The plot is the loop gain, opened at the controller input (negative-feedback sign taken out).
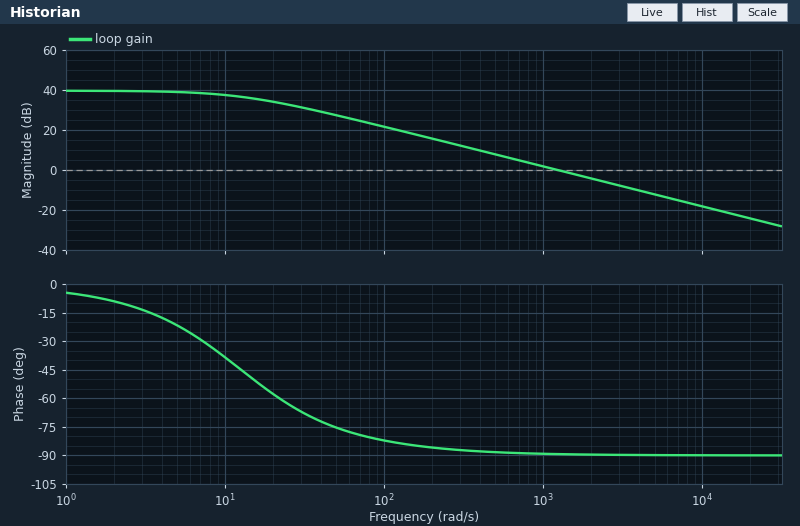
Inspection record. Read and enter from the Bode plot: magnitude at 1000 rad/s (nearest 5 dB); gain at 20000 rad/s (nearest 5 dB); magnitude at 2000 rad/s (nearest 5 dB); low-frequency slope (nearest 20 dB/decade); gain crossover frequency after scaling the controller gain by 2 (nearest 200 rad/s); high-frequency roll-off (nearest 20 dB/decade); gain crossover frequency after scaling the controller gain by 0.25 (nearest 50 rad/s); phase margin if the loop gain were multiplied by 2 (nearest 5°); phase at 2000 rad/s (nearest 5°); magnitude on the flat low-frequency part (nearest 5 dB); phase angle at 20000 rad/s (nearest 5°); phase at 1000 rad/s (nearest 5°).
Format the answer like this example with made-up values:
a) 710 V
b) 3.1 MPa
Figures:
a) 0 dB
b) -25 dB
c) -5 dB
d) 0 dB/decade
e) 2400 rad/s
f) -20 dB/decade
g) 300 rad/s
h) 90°
i) -90°
j) 40 dB
k) -90°
l) -90°
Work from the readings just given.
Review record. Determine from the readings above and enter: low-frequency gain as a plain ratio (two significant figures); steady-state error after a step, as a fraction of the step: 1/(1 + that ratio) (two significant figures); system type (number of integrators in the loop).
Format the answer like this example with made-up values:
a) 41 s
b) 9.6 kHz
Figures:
a) 100
b) 0.0099
c) 0
